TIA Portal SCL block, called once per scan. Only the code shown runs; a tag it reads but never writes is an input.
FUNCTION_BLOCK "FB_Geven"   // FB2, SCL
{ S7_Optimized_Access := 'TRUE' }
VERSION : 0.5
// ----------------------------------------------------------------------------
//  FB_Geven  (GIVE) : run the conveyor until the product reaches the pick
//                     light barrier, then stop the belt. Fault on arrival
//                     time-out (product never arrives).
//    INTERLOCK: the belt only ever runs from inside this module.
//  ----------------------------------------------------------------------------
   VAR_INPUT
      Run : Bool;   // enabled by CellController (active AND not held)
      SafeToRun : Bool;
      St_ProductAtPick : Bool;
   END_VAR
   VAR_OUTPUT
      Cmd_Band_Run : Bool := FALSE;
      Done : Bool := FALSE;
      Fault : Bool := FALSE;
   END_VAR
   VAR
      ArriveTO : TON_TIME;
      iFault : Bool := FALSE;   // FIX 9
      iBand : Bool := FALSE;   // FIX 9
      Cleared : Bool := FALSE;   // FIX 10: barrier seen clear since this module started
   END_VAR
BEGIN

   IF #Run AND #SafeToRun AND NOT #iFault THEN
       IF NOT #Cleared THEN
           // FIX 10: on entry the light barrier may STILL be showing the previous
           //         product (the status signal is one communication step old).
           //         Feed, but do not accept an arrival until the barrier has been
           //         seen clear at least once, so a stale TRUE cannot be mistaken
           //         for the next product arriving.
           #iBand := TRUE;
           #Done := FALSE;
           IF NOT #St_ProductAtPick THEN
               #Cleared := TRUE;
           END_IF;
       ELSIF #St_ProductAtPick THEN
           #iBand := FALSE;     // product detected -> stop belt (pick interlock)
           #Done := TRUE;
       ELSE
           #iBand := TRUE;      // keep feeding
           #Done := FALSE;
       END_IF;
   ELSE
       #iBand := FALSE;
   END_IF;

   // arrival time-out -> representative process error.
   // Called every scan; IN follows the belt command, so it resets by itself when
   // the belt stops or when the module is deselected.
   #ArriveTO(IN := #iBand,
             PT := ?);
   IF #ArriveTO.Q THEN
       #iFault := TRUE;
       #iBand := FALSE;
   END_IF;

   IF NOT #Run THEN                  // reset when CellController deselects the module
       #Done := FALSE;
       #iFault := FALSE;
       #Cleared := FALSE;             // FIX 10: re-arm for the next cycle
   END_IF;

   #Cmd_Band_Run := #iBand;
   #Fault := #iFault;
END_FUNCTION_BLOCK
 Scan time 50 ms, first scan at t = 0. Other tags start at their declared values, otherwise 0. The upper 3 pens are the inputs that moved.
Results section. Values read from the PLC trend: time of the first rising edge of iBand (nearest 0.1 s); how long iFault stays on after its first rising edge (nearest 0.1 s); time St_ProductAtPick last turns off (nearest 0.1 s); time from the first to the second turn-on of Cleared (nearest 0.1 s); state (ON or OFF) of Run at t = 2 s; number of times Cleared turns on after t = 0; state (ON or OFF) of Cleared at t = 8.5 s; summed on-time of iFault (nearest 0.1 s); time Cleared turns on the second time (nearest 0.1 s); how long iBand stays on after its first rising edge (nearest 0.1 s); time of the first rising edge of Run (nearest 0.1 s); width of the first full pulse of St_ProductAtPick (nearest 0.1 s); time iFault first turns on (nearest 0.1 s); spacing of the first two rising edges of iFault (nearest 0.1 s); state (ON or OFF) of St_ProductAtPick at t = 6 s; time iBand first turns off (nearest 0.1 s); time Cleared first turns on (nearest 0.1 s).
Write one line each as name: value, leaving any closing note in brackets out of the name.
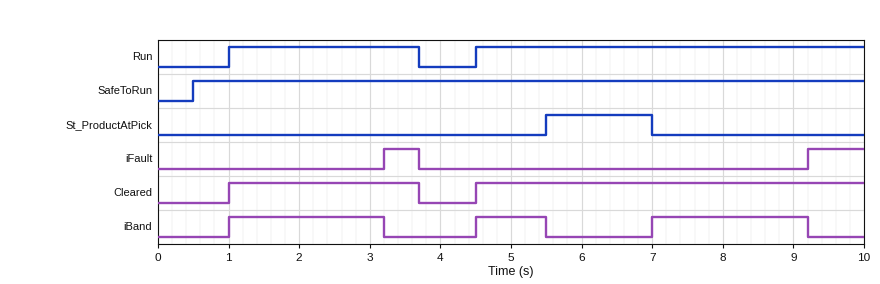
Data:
time of the first rising edge of iBand: 1.0 s
how long iFault stays on after its first rising edge: 0.5 s
time St_ProductAtPick last turns off: 7.0 s
time from the first to the second turn-on of Cleared: 3.5 s
state (ON or OFF) of Run at t = 2 s: ON
number of times Cleared turns on after t = 0: 2
state (ON or OFF) of Cleared at t = 8.5 s: ON
summed on-time of iFault: 1.3 s
time Cleared turns on the second time: 4.5 s
how long iBand stays on after its first rising edge: 2.2 s
time of the first rising edge of Run: 1.0 s
width of the first full pulse of St_ProductAtPick: 1.5 s
time iFault first turns on: 3.2 s
spacing of the first two rising edges of iFault: 6.0 s
state (ON or OFF) of St_ProductAtPick at t = 6 s: ON
time iBand first turns off: 3.2 s
time Cleared first turns on: 1.0 s
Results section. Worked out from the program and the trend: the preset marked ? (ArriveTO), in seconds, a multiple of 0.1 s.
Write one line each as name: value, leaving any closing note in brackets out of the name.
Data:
the preset marked ? (ArriveTO), in seconds, a multiple of 0.1 s: 2.2 s
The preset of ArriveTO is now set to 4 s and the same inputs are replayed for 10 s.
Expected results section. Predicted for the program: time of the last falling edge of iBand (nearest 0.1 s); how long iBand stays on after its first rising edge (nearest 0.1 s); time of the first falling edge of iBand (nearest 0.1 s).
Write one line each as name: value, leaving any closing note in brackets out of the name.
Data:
time of the last falling edge of iBand: 5.5 s
how long iBand stays on after its first rising edge: 2.7 s
time of the first falling edge of iBand: 3.7 s
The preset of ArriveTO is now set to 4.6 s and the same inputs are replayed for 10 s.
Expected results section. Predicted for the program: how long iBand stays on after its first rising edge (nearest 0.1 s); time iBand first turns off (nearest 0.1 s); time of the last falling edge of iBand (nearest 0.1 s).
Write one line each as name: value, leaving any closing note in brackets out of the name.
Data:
how long iBand stays on after its first rising edge: 2.7 s
time iBand first turns off: 3.7 s
time of the last falling edge of iBand: 5.5 s
